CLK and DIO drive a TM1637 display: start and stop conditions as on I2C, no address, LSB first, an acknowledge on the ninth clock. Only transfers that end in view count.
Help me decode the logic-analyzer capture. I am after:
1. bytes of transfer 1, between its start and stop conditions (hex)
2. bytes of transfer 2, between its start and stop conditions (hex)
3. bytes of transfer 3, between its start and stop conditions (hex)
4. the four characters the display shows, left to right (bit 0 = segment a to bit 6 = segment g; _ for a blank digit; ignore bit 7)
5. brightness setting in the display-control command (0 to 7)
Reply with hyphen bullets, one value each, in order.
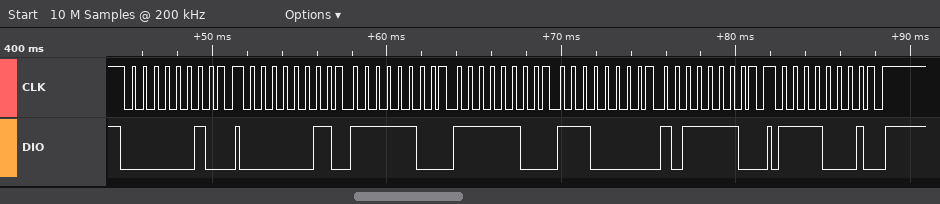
- 40
- C0 3F 3F 07 7D
- 8F
- 0076
- 7
